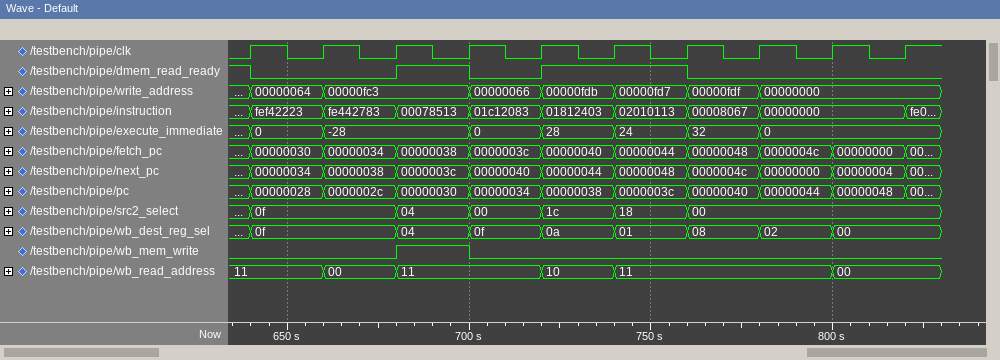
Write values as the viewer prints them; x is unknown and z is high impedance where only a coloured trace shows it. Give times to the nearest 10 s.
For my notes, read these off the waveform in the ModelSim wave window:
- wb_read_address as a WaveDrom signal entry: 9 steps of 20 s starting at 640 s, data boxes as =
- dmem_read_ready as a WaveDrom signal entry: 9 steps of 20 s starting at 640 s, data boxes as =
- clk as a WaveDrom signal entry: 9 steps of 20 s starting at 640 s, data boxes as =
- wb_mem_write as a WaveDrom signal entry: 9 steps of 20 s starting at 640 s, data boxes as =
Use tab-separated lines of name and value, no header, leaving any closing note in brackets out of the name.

wb_read_address as a WaveDrom signal entry: 9 steps of 20 s starting at 640 s, data boxes as =	{name: 'wb_read_address', wave: '===.==..=', data: '11 00 11 10 11 00'}
dmem_read_ready as a WaveDrom signal entry: 9 steps of 20 s starting at 640 s, data boxes as =	{name: 'dmem_read_ready', wave: '0.101.0..'}
clk as a WaveDrom signal entry: 9 steps of 20 s starting at 640 s, data boxes as =	{name: 'clk', wave: 'p........'}
wb_mem_write as a WaveDrom signal entry: 9 steps of 20 s starting at 640 s, data boxes as =	{name: 'wb_mem_write', wave: '0.10.....'}
